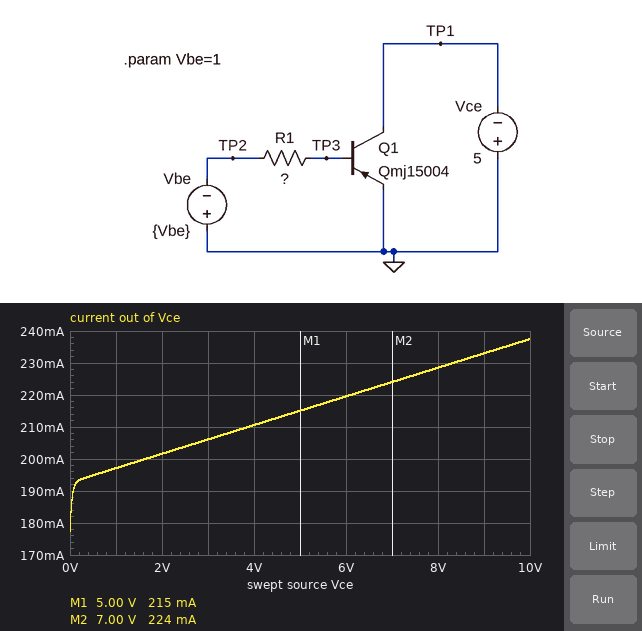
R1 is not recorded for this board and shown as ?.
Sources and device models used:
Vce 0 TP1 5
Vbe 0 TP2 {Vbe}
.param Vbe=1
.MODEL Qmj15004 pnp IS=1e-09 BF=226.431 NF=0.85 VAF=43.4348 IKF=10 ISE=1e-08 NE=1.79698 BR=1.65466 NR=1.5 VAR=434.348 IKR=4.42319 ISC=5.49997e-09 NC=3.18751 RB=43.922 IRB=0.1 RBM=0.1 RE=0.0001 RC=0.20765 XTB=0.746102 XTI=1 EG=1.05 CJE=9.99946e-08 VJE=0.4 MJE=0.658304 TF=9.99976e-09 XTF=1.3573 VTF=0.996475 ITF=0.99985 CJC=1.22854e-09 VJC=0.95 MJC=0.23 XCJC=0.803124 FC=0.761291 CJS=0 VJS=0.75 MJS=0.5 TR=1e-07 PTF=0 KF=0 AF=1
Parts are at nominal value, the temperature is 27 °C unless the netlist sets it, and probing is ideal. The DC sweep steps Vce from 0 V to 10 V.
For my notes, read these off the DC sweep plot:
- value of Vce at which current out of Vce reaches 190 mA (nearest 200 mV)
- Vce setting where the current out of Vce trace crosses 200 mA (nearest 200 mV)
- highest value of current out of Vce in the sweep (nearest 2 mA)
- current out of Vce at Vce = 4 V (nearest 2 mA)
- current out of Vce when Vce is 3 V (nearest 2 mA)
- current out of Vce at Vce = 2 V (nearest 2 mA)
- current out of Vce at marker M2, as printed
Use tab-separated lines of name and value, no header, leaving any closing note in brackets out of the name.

value of Vce at which current out of Vce reaches 190 mA	0 V
Vce setting where the current out of Vce trace crosses 200 mA	1.6 V
highest value of current out of Vce in the sweep	238 mA
current out of Vce at Vce = 4 V	210 mA
current out of Vce when Vce is 3 V	206 mA
current out of Vce at Vce = 2 V	202 mA
current out of Vce at marker M2, as printed	224 mA
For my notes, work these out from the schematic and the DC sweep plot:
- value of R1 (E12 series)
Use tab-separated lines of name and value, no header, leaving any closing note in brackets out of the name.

value of R1	560 Ω
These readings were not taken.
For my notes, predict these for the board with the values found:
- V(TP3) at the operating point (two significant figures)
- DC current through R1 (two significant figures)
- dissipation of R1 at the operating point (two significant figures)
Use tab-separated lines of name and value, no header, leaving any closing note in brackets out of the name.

V(TP3) at the operating point	-460 mV
DC current through R1	960 µA
dissipation of R1 at the operating point	520 µW
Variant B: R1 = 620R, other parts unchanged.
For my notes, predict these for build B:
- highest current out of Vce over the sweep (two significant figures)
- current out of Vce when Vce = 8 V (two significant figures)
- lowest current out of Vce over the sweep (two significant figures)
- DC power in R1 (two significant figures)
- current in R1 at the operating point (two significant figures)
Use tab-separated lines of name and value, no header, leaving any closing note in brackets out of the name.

highest current out of Vce over the sweep	220 mA
current out of Vce when Vce = 8 V	210 mA
lowest current out of Vce over the sweep	160 mA
DC power in R1	480 µW
current in R1 at the operating point	880 µA
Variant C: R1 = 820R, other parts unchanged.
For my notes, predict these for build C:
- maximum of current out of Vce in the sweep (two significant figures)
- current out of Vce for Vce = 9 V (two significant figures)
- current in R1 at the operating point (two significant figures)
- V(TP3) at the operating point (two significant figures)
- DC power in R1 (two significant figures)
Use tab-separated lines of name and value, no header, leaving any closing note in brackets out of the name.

maximum of current out of Vce in the sweep	170 mA
current out of Vce for Vce = 9 V	160 mA
current in R1 at the operating point	680 µA
V(TP3) at the operating point	-440 mV
DC power in R1	380 µW
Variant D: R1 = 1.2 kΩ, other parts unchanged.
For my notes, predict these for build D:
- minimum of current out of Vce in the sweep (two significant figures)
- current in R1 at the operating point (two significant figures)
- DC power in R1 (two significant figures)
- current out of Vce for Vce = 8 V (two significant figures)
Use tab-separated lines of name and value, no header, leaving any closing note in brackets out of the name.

minimum of current out of Vce in the sweep	87 mA
current in R1 at the operating point	480 µA
DC power in R1	280 µW
current out of Vce for Vce = 8 V	110 mA
